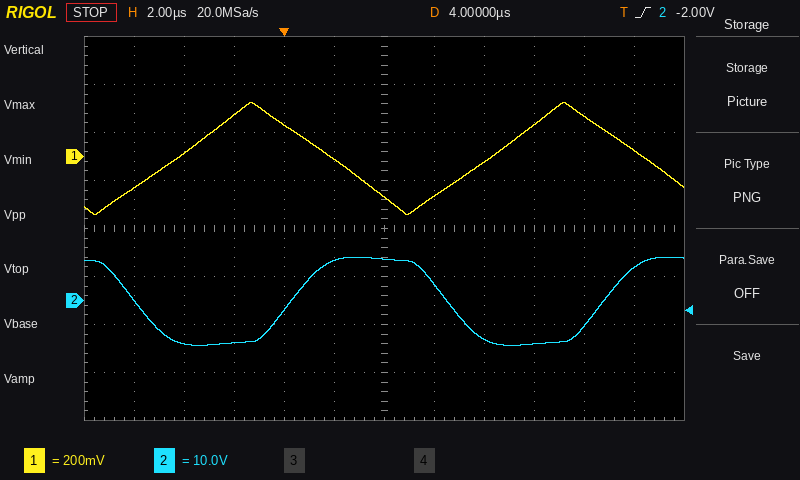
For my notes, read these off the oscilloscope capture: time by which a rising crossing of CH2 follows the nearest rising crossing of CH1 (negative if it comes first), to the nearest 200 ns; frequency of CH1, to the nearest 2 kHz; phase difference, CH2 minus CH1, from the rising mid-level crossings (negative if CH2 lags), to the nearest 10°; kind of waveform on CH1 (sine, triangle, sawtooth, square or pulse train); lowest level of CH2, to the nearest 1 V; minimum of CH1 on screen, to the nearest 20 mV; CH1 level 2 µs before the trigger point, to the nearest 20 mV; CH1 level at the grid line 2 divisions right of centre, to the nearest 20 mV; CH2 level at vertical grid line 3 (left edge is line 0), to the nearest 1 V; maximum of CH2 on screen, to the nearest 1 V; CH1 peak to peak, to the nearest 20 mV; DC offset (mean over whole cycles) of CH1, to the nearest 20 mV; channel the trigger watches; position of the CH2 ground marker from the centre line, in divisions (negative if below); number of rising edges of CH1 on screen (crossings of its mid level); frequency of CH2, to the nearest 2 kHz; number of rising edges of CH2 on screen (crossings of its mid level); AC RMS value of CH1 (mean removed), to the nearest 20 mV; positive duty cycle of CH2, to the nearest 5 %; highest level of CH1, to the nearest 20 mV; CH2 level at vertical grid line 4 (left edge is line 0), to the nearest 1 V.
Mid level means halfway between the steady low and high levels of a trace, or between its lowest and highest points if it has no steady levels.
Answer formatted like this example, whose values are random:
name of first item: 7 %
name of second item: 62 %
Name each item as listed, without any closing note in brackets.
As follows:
time by which a rising crossing of CH2 follows the nearest rising crossing of CH1 (negative if it comes first), to the nearest 200 ns: +4.6 µs
frequency of CH1, to the nearest 2 kHz: 80 kHz
phase difference, CH2 minus CH1, from the rising mid-level crossings (negative if CH2 lags), to the nearest 10°: -130°
kind of waveform on CH1: triangle
lowest level of CH2, to the nearest 1 V: -9 V
minimum of CH1 on screen, to the nearest 20 mV: -240 mV
CH1 level 2 µs before the trigger point, to the nearest 20 mV: 180 mV
CH1 level at the grid line 2 divisions right of centre, to the nearest 20 mV: -20 mV
CH2 level at vertical grid line 3 (left edge is line 0), to the nearest 1 V: -9 V
maximum of CH2 on screen, to the nearest 1 V: 9 V
CH1 peak to peak, to the nearest 20 mV: 460 mV
DC offset (mean over whole cycles) of CH1, to the nearest 20 mV: 0 mV
channel the trigger watches: CH2
position of the CH2 ground marker from the centre line, in divisions: -1.5 div
number of rising edges of CH1 on screen: 2
frequency of CH2, to the nearest 2 kHz: 80 kHz
number of rising edges of CH2 on screen: 2
AC RMS value of CH1 (mean removed), to the nearest 20 mV: 140 mV
positive duty cycle of CH2, to the nearest 5 %: 50 %
highest level of CH1, to the nearest 20 mV: 220 mV
CH2 level at vertical grid line 4 (left edge is line 0), to the nearest 1 V: -2 V
